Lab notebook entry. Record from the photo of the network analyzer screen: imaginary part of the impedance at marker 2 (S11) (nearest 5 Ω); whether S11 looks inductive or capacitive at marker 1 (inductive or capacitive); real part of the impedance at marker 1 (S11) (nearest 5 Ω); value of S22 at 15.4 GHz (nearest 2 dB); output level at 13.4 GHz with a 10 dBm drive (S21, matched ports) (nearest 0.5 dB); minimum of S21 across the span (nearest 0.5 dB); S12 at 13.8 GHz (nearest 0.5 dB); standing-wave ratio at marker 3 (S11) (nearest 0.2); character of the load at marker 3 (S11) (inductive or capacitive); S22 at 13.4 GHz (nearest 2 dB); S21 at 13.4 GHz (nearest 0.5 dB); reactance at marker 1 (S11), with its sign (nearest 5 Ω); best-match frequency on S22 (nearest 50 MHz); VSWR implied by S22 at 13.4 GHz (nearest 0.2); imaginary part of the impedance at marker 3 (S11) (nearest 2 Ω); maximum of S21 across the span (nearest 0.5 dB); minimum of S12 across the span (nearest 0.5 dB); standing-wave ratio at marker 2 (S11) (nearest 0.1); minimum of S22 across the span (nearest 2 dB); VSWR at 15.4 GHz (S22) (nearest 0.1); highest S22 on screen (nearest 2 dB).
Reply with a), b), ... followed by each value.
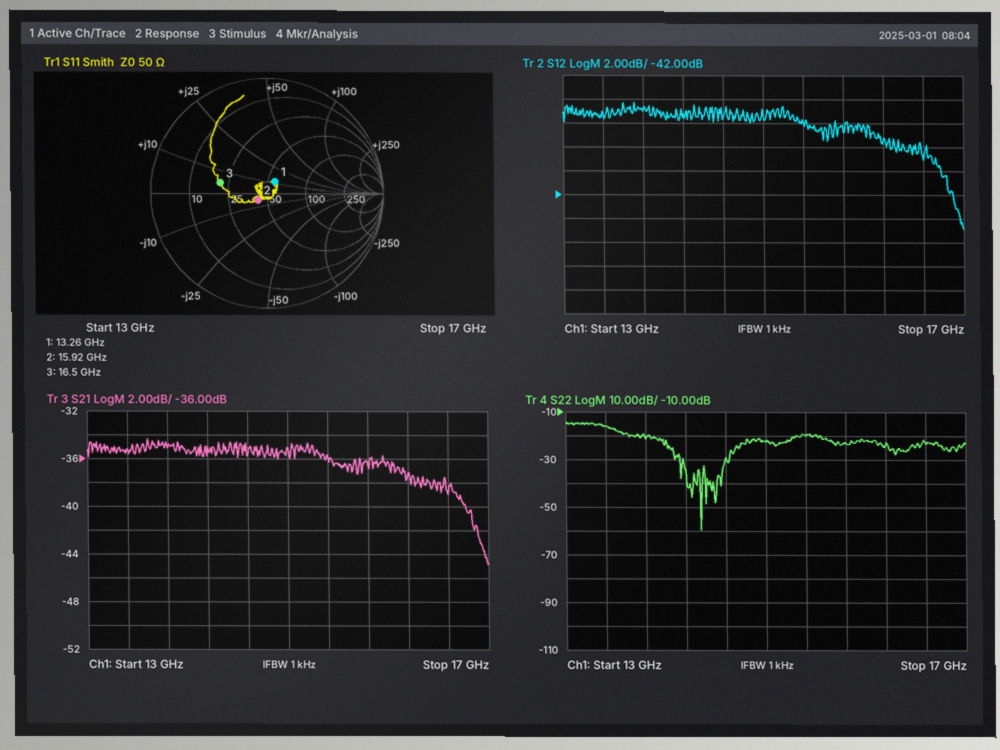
a) -5 Ω
b) inductive
c) 55 Ω
d) -20 dB
e) -25.5 dBm
f) -45.0 dB
g) -35.0 dB
h) 2.4
i) inductive
j) -16 dB
k) -35.5 dB
l) +10 Ω
m) 14.35 GHz
n) 1.4
o) +4 Ω
p) -34.5 dB
q) -45.0 dB
r) 1.2
s) -60 dB
t) 1.2
u) -14 dB
